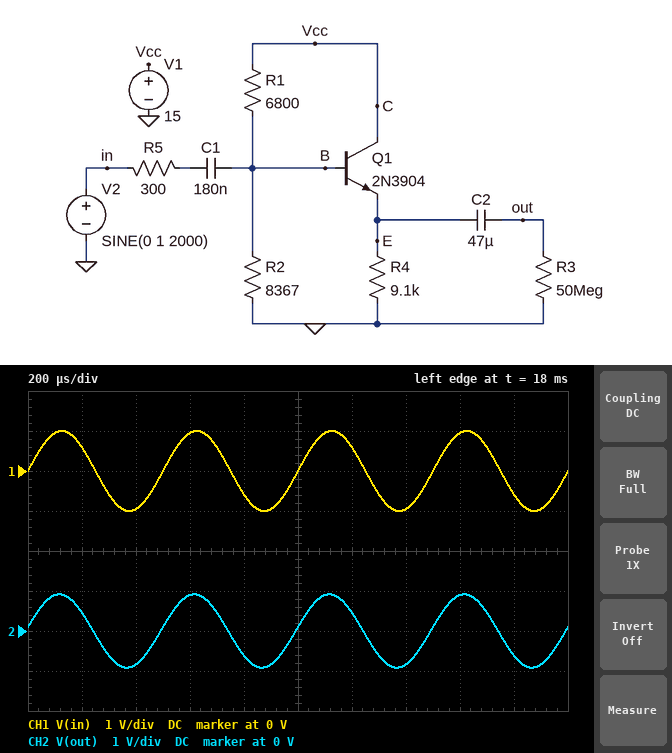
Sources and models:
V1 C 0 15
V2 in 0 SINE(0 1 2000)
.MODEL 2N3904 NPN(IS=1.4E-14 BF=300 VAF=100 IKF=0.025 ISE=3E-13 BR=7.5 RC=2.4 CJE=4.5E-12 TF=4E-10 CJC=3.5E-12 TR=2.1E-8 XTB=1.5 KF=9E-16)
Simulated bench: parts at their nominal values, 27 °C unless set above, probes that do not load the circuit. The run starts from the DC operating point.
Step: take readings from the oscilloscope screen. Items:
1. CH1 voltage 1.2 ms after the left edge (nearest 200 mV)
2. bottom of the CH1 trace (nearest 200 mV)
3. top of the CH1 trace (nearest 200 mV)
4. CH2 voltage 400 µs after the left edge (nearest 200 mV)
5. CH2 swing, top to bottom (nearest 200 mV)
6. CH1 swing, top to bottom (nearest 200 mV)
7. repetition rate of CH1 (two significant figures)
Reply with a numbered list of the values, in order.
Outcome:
1. 600 mV
2. -1.0 V
3. 1.0 V
4. -800 mV
5. 1.8 V
6. 2.0 V
7. 2.0 kHz
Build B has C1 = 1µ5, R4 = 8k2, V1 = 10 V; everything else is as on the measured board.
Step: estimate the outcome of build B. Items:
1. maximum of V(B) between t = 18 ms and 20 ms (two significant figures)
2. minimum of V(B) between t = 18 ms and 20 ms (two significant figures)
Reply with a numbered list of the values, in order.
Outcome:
1. 6.4 V
2. 4.6 V
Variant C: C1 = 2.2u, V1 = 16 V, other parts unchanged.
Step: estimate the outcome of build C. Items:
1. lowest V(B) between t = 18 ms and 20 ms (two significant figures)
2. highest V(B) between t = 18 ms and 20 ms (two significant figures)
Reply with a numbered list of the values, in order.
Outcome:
1. 7.9 V
2. 9.7 V
